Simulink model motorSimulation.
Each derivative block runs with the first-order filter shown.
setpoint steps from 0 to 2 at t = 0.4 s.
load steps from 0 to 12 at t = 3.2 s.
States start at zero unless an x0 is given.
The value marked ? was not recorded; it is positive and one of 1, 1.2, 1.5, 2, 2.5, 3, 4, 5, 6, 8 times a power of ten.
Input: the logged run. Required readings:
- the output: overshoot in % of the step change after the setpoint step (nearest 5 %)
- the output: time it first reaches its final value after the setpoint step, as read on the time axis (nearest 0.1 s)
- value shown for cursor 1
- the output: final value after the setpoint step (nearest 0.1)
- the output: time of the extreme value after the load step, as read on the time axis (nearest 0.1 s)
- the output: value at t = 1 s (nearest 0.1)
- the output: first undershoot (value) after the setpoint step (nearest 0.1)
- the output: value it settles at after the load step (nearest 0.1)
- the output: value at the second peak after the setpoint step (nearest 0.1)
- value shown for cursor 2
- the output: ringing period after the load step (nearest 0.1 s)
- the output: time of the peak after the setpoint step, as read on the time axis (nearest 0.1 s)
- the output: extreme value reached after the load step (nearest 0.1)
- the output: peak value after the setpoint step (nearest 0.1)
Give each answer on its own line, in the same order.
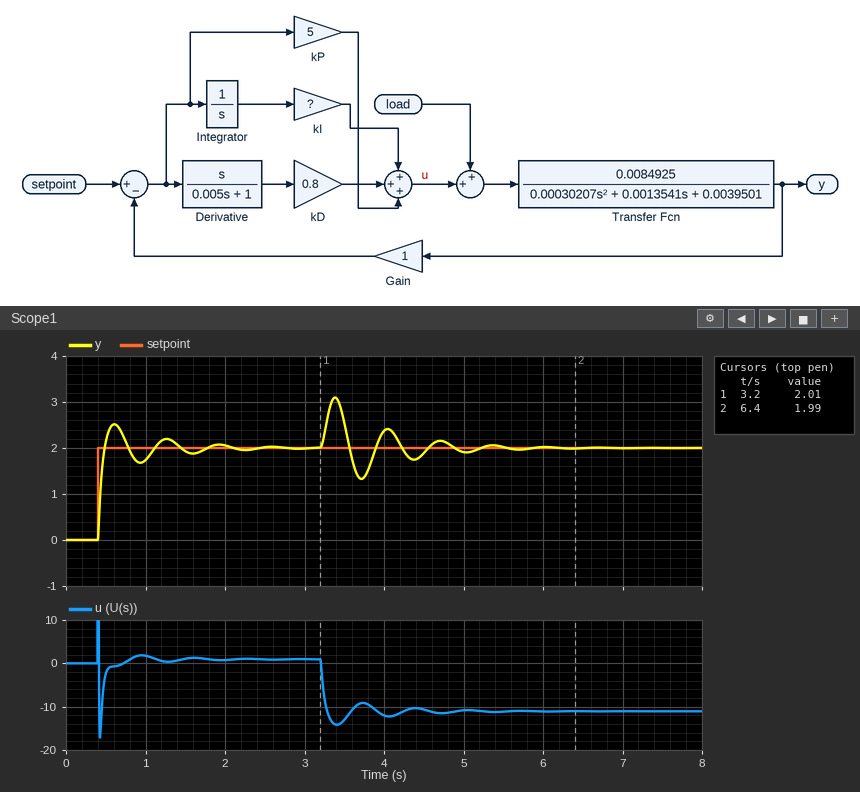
25 %
0.5 s
2.01
2.0
3.4 s
1.7
1.7
2.0
2.2
1.99
0.7 s
0.6 s
3.1
2.5
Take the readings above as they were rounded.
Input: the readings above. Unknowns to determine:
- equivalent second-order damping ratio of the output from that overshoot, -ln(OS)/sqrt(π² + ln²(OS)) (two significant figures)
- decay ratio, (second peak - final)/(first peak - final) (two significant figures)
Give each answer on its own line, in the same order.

0.40
0.40
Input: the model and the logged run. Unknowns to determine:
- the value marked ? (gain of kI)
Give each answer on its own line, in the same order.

80
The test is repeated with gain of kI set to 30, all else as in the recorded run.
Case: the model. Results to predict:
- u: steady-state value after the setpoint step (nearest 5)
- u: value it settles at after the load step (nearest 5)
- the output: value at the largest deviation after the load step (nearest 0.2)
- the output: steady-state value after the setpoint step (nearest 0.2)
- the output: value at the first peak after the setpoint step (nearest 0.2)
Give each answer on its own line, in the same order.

0
-10
3.4
2.0
2.2
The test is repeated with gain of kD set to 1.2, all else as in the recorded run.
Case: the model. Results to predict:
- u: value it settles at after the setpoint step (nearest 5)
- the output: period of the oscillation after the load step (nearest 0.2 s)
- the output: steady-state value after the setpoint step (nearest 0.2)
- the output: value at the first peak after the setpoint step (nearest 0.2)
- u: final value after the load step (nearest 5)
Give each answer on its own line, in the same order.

0
0.8 s
2.0
2.2
-10
